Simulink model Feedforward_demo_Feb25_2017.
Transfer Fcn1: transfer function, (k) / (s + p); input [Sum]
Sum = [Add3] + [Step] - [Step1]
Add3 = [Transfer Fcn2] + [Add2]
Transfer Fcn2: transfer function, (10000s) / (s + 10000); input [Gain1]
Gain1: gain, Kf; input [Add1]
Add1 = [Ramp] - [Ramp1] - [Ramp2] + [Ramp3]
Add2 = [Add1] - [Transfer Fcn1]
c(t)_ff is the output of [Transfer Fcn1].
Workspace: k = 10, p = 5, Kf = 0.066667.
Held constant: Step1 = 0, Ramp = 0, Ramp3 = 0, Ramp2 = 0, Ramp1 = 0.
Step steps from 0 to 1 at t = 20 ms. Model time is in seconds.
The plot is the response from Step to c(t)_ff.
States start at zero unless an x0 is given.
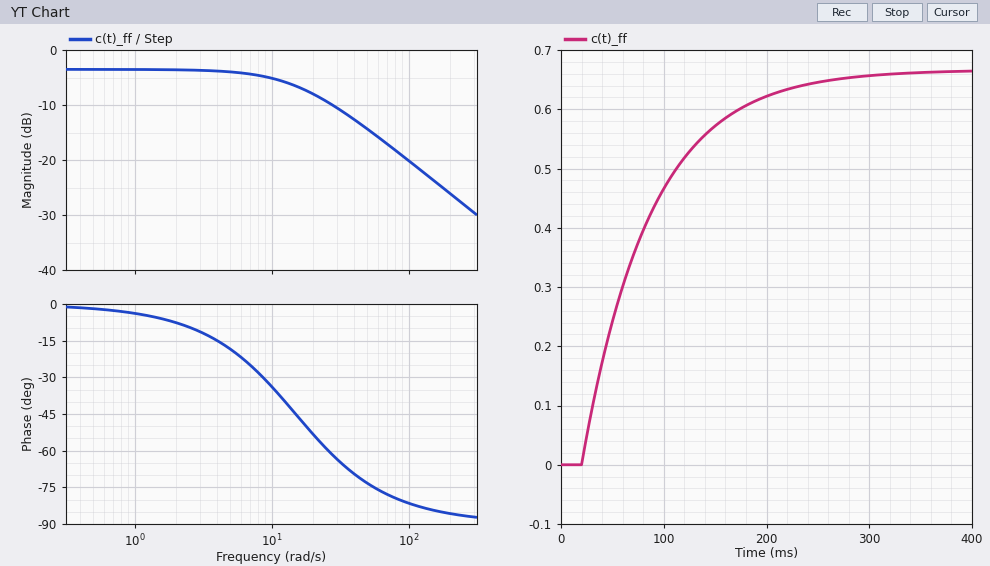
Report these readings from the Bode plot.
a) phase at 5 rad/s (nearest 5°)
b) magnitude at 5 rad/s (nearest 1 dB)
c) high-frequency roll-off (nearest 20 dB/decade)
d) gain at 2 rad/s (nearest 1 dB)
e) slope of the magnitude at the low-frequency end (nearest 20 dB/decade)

-20°
-4 dB
-20 dB/decade
-4 dB
0 dB/decade
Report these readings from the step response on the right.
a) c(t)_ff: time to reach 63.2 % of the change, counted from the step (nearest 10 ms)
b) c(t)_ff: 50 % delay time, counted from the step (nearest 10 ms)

70 ms
50 ms
